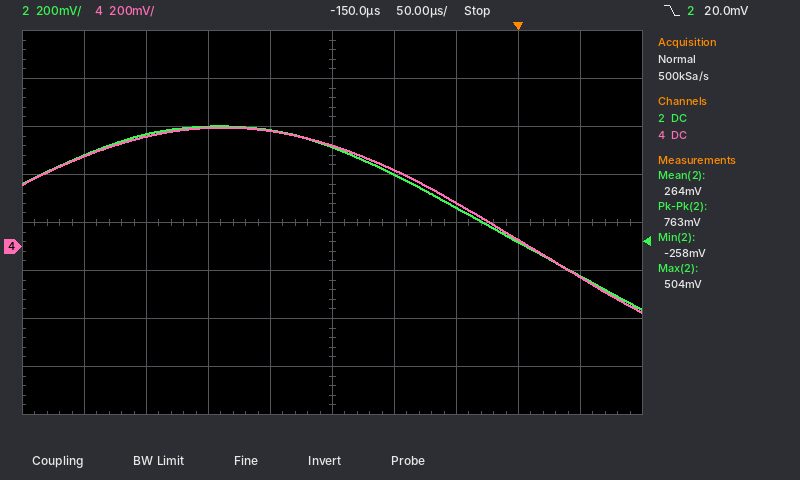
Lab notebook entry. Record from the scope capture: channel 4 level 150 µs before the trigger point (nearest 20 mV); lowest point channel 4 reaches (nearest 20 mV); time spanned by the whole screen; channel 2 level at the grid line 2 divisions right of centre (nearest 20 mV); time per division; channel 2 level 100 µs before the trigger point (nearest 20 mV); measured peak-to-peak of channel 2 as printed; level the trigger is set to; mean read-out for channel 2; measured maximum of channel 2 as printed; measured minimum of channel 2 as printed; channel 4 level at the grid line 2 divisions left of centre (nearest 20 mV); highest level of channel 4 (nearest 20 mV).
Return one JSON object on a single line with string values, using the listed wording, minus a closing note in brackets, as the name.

{"channel 4 level 150 µs before the trigger point": "420 mV", "lowest point channel 4 reaches": "-280 mV", "time spanned by the whole screen": "500 µs", "channel 2 level at the grid line 2 divisions right of centre": "160 mV", "time per division": "50 µs", "channel 2 level 100 µs before the trigger point": "300 mV", "measured peak-to-peak of channel 2 as printed": "763 mV", "level the trigger is set to": "20.0 mV", "mean read-out for channel 2": "264 mV", "measured maximum of channel 2 as printed": "504 mV", "measured minimum of channel 2 as printed": "-258 mV", "channel 4 level at the grid line 2 divisions left of centre": "500 mV", "highest level of channel 4": "500 mV"}
